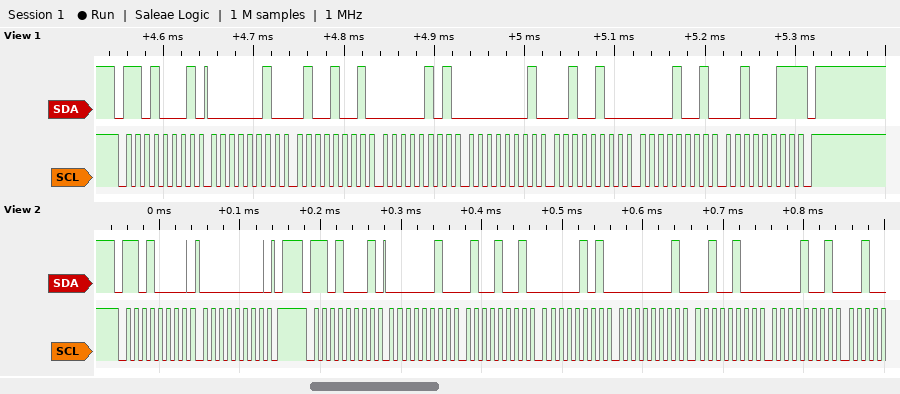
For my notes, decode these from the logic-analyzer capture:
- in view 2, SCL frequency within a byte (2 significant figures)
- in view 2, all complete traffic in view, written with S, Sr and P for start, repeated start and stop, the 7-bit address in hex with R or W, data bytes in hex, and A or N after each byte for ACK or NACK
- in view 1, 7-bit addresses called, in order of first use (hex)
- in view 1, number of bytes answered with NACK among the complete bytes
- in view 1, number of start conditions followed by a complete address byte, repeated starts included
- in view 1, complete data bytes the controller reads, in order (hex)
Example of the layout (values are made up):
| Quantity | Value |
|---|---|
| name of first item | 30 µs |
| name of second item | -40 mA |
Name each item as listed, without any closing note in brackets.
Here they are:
| Quantity | Value |
|---|---|
| in view 2, SCL frequency within a byte | 100 kHz |
| in view 2, all complete traffic in view, written with S, Sr and P for start, repeated start and stop, the 7-bit address in hex with R or W, data bytes in hex, and A or N after each byte for ACK or NACK | S 68W A 00 A P S 68R A 02 A 49 A 05 A 01 A 24 A 09 A |
| in view 1, 7-bit addresses called, in order of first use | 0x68 |
| in view 1, number of bytes answered with NACK among the complete bytes | 1 |
| in view 1, number of start conditions followed by a complete address byte, repeated starts included | 1 |
| in view 1, complete data bytes the controller reads, in order | 02 49 05 01 24 09 23 |
